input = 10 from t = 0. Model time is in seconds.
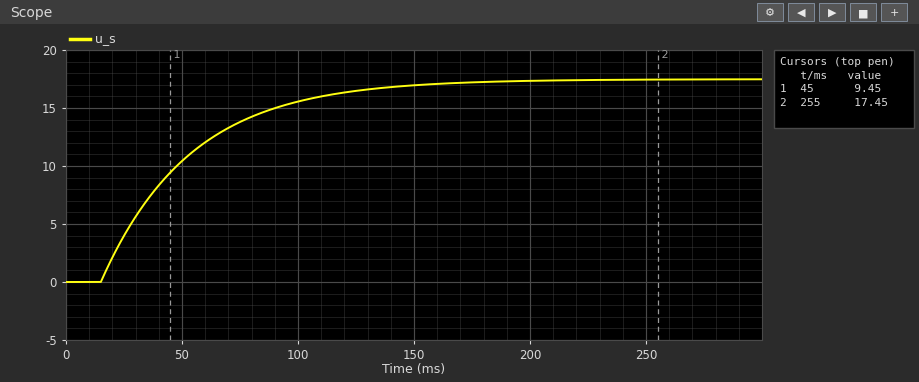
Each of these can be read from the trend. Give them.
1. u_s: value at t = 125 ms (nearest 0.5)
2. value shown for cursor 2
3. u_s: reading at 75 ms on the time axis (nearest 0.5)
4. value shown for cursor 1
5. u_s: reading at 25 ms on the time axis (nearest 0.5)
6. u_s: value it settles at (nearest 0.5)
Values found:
16.5
17.45
14.0
9.45
4.0
17.5
